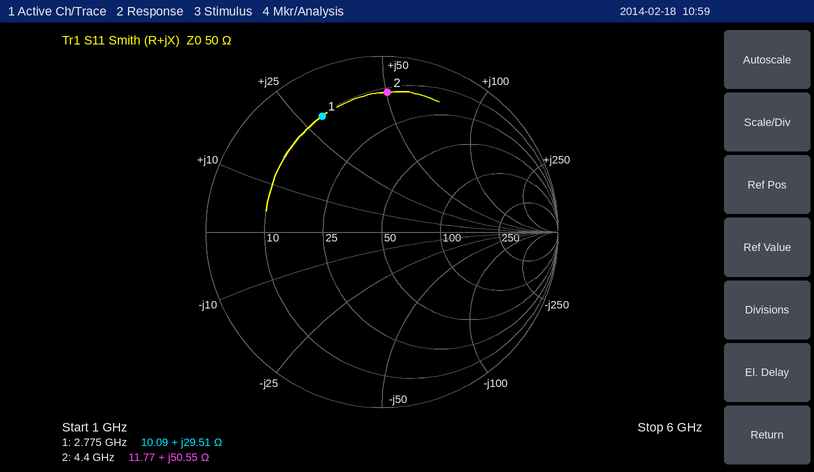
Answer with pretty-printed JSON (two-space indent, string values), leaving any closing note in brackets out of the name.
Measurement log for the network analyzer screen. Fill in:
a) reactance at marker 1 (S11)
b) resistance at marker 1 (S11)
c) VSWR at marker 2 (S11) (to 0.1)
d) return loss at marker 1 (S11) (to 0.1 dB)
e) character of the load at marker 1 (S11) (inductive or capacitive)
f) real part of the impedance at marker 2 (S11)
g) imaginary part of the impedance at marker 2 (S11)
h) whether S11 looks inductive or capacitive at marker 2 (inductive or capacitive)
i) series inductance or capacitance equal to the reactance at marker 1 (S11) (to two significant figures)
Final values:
{
  "reactance at marker 1": "+29.51 Ω",
  "resistance at marker 1": "10.09 Ω",
  "VSWR at marker 2 (S11)": "8.7",
  "return loss at marker 1 (S11)": "2.6 dB",
  "character of the load at marker 1 (S11)": "inductive",
  "real part of the impedance at marker 2": "11.77 Ω",
  "imaginary part of the impedance at marker 2": "+50.55 Ω",
  "whether S11 looks inductive or capacitive at marker 2": "inductive",
  "series inductance or capacitance equal to the reactance at marker 1 (S11)": "1.7 nH"
}
